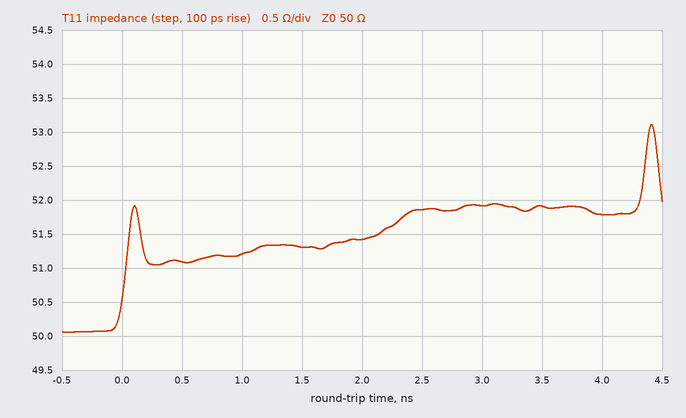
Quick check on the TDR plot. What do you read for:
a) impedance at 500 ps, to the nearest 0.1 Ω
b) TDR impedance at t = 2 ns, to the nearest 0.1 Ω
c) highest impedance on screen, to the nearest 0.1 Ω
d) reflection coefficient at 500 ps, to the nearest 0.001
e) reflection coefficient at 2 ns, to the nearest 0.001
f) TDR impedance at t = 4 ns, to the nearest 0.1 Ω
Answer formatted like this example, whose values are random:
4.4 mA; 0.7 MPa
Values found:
51.1 Ω; 51.4 Ω; 53.1 Ω; +0.011; +0.014; 51.8 Ω
